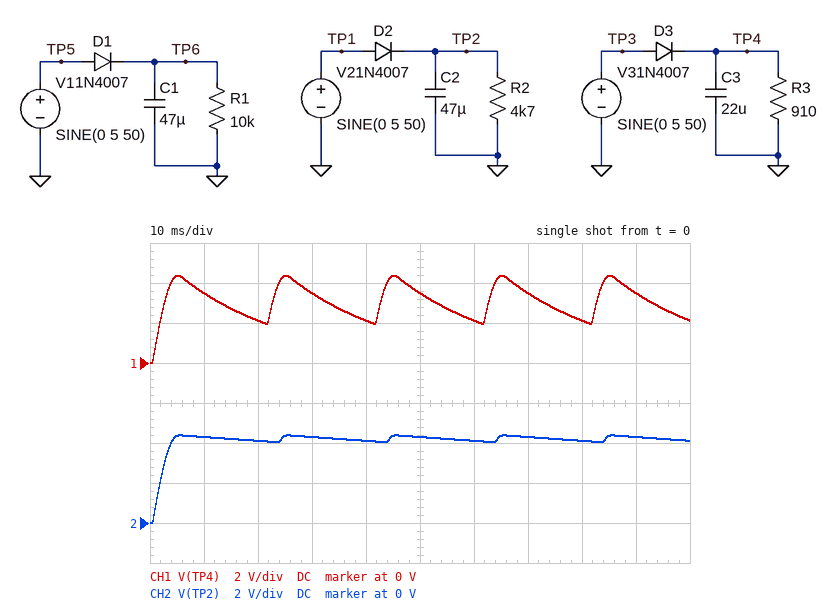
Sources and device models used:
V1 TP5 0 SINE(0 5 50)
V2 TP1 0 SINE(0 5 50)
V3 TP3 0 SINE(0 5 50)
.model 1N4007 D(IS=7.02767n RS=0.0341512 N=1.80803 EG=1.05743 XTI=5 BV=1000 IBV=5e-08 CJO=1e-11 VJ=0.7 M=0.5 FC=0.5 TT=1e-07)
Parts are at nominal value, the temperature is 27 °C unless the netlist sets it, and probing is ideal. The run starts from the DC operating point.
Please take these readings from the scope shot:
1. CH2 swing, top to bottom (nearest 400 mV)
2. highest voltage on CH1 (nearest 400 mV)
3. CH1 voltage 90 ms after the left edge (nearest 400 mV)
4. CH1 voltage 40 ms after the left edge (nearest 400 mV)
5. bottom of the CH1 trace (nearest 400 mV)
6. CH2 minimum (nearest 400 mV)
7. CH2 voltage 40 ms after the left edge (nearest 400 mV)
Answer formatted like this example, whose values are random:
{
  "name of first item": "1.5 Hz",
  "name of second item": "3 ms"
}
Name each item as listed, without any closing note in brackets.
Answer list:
{
  "CH2 swing, top to bottom": "4.4 V",
  "highest voltage on CH1": "4.4 V",
  "CH1 voltage 90 ms after the left edge": "3.6 V",
  "CH1 voltage 40 ms after the left edge": "2.0 V",
  "bottom of the CH1 trace": "0 V",
  "CH2 minimum": "0 V",
  "CH2 voltage 40 ms after the left edge": "4.0 V"
}
